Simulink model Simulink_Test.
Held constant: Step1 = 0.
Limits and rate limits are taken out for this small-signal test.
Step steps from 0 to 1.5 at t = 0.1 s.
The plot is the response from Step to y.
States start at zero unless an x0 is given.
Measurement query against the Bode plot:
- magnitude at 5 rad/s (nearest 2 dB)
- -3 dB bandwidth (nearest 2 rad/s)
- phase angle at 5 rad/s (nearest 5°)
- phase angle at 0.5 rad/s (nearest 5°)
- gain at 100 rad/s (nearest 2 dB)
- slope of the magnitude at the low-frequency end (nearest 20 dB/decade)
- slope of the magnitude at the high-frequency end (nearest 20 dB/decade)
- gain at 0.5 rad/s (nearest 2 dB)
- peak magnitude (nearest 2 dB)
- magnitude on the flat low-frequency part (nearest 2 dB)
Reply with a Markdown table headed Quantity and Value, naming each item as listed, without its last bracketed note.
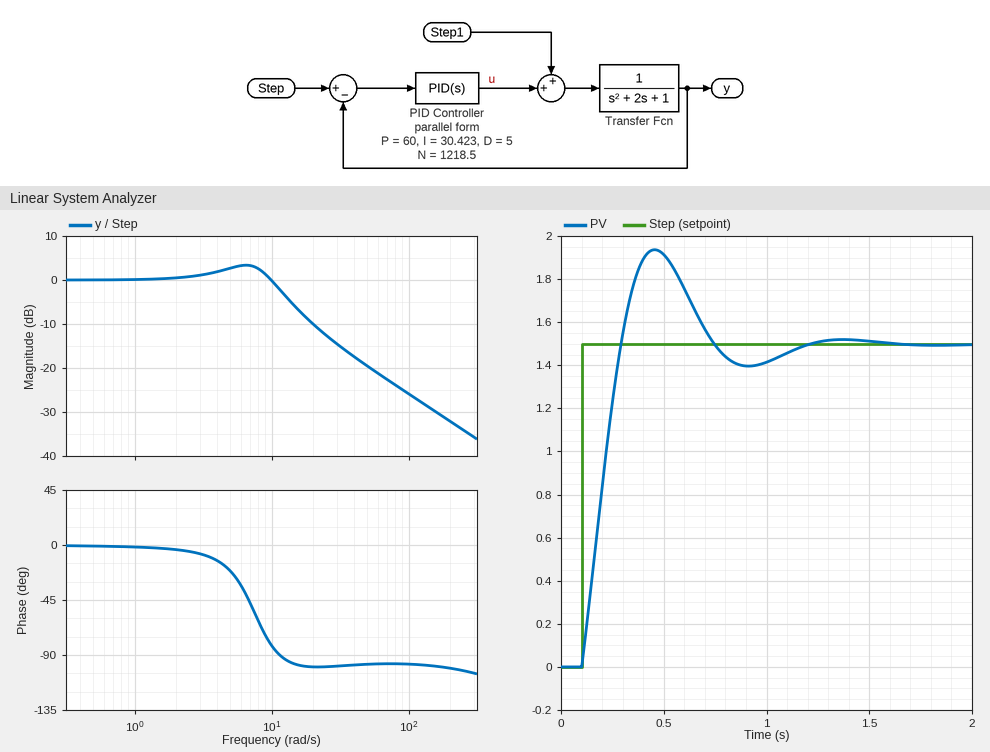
| Quantity | Value |
|---|---|
| magnitude at 5 rad/s | 2 dB |
| -3 dB bandwidth | 12 rad/s |
| phase angle at 5 rad/s | -20° |
| phase angle at 0.5 rad/s | 0° |
| gain at 100 rad/s | -26 dB |
| slope of the magnitude at the low-frequency end | 0 dB/decade |
| slope of the magnitude at the high-frequency end | -20 dB/decade |
| gain at 0.5 rad/s | 0 dB |
| peak magnitude | 4 dB |
| magnitude on the flat low-frequency part | 0 dB |
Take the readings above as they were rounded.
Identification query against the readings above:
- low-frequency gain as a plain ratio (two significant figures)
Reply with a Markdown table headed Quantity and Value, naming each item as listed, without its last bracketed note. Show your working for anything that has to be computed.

| Quantity | Value |
|---|---|
| low-frequency gain as a plain ratio | 10^(0 / 20) = 1.0 |
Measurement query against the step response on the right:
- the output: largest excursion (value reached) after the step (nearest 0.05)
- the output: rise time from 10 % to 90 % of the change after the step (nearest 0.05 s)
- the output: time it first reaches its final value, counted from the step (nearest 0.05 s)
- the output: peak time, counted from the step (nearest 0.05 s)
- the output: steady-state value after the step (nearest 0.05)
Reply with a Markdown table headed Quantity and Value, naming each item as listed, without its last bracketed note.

| Quantity | Value |
|---|---|
| the output: largest excursion (value reached) after the step | 1.95 |
| the output: rise time from 10 % to 90 % of the change after the step | 0.15 s |
| the output: time it first reaches its final value, counted from the step | 0.20 s |
| the output: peak time, counted from the step | 0.35 s |
| the output: steady-state value after the step | 1.50 |
